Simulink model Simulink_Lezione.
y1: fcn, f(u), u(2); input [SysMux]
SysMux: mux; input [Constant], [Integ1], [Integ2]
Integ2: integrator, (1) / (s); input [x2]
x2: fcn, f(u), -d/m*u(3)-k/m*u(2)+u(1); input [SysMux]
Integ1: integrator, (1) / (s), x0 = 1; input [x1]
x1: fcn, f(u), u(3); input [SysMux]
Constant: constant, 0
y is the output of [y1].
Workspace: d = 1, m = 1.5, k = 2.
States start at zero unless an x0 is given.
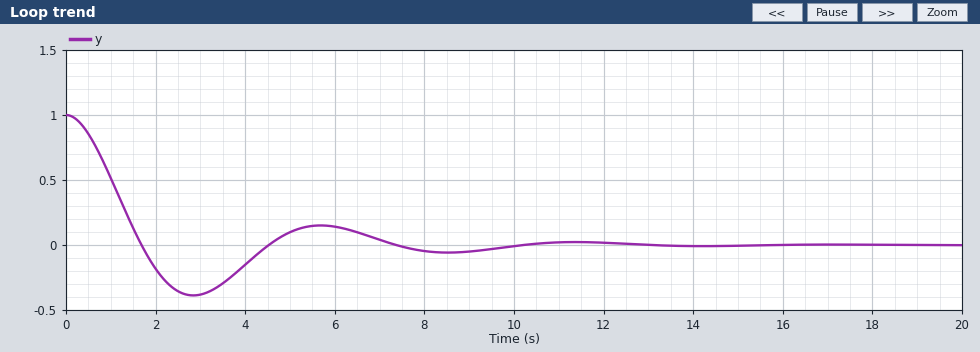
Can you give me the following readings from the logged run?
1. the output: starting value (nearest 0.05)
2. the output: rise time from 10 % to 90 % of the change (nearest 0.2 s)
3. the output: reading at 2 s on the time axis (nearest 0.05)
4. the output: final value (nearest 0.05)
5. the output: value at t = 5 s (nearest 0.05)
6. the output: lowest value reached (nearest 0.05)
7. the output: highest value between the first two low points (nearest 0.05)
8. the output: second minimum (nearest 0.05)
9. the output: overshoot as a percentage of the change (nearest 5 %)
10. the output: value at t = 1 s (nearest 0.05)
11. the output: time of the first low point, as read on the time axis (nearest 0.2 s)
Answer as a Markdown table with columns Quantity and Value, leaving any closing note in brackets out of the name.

| Quantity | Value |
|---|---|
| the output: starting value | 1.00 |
| the output: rise time from 10 % to 90 % of the change | 1.2 s |
| the output: reading at 2 s on the time axis | -0.20 |
| the output: final value | 0.00 |
| the output: value at t = 5 s | 0.10 |
| the output: lowest value reached | -0.40 |
| the output: highest value between the first two low points | 0.15 |
| the output: second minimum | -0.05 |
| the output: overshoot as a percentage of the change | 40 % |
| the output: value at t = 1 s | 0.50 |
| the output: time of the first low point, as read on the time axis | 2.8 s |
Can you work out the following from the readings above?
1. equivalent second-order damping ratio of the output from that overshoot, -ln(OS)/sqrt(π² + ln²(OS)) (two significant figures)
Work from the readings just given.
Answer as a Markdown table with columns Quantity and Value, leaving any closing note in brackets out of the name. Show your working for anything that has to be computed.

| Quantity | Value |
|---|---|
| equivalent second-order damping ratio of the output from that overshoot, -ln(OS)/sqrt(π² + ln²(OS)) | ln(0.4) = -0.916; 0.916 / sqrt(9.870 + 0.840) = 0.28 |
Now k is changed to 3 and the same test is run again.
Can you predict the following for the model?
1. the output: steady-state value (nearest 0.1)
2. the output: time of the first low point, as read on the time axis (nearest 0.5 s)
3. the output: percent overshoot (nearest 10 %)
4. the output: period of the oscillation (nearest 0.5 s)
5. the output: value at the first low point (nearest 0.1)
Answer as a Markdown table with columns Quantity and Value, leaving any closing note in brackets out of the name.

| Quantity | Value |
|---|---|
| the output: steady-state value | 0.0 |
| the output: time of the first low point, as read on the time axis | 2.5 s |
| the output: percent overshoot | 50 % |
| the output: period of the oscillation | 4.5 s |
| the output: value at the first low point | -0.5 |
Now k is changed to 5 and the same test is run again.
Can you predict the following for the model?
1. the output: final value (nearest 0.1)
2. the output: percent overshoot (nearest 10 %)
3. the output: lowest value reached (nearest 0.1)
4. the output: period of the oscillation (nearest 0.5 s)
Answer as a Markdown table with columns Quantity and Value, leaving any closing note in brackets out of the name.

| Quantity | Value |
|---|---|
| the output: final value | 0.0 |
| the output: percent overshoot | 60 % |
| the output: lowest value reached | -0.6 |
| the output: period of the oscillation | 3.5 s |
